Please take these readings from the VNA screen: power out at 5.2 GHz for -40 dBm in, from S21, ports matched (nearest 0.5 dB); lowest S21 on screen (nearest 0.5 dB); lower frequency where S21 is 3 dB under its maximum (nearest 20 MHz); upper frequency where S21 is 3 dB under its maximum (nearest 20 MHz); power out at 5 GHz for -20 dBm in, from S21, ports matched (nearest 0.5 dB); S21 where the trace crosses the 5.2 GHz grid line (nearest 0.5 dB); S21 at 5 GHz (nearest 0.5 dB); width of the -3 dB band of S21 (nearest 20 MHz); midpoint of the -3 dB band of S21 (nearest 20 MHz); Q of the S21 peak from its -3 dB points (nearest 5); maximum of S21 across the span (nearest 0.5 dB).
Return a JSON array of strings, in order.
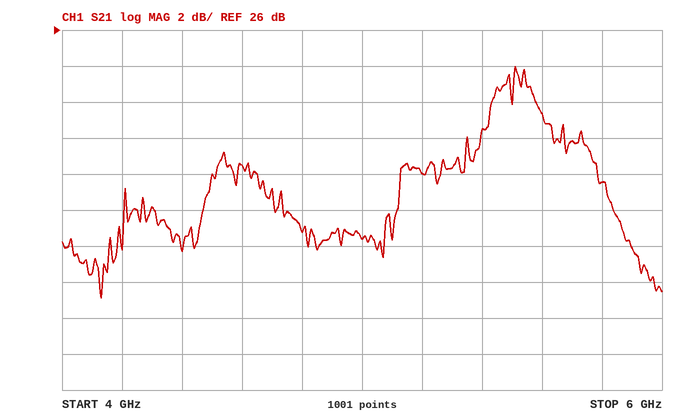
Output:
["-22.0 dBm", "11.0 dB", "5.42 GHz", "5.60 GHz", "-5.5 dBm", "18.0 dB", "14.5 dB", "180 MHz", "5.52 GHz", "30", "24.0 dB"]
